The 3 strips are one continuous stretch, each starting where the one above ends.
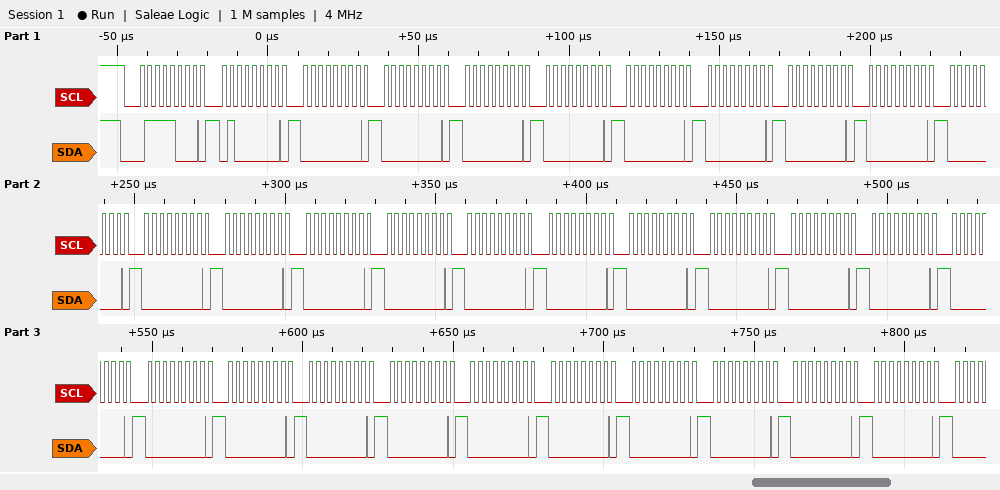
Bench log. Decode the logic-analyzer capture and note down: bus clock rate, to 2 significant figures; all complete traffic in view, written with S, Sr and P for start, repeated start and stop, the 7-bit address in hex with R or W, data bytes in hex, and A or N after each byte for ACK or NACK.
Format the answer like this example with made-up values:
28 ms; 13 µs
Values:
400 kHz; S 3CW A 40 A 00 A 00 A 00 A 00 A 00 A 00 A 00 A 00 A 00 A 00 A 00 A 00 A 00 A 00 A 00 A 00 A 00 A 00 A 00 A 00 A 00 A 00 A 00 A 00 A 00 A 00 A 00 A 00 A 00 A 00 A
